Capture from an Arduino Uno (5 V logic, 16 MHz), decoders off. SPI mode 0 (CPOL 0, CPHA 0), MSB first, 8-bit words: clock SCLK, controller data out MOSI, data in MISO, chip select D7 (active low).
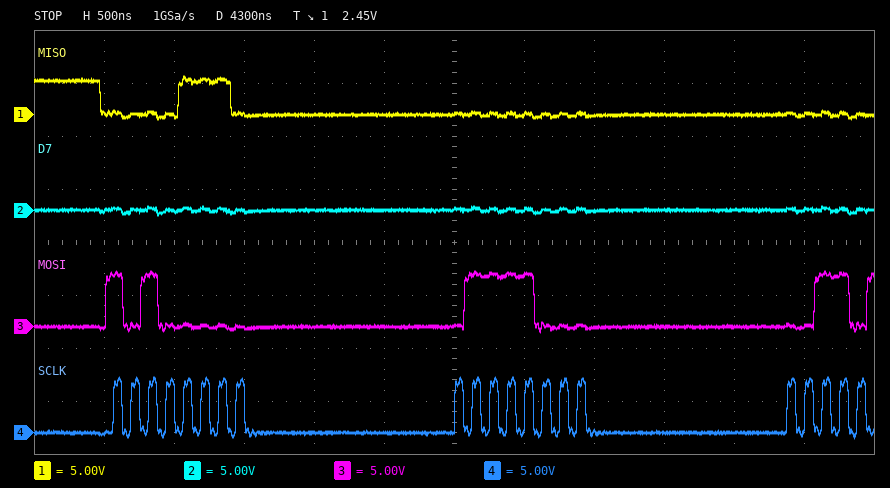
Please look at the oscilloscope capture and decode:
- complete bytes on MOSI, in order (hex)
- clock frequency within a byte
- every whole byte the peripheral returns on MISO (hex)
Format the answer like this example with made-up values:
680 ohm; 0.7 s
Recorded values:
A0 78; 8 MHz; 0E 00
